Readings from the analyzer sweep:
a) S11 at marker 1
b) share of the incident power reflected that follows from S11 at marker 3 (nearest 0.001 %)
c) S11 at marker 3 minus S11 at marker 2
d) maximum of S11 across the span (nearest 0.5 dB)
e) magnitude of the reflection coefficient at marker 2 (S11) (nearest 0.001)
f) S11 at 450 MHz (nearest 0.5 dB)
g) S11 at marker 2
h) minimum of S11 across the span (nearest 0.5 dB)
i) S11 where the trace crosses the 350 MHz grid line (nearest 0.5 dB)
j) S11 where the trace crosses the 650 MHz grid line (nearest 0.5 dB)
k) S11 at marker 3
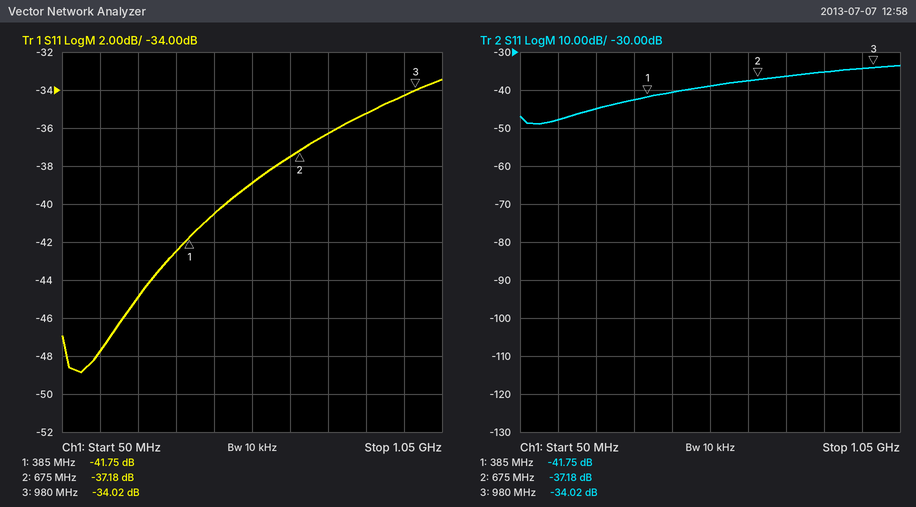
-41.75 dB
0.040 %
3.16 dB
-33.5 dB
0.014
-40.5 dB
-37.18 dB
-49.0 dB
-42.5 dB
-37.5 dB
-34.02 dB
